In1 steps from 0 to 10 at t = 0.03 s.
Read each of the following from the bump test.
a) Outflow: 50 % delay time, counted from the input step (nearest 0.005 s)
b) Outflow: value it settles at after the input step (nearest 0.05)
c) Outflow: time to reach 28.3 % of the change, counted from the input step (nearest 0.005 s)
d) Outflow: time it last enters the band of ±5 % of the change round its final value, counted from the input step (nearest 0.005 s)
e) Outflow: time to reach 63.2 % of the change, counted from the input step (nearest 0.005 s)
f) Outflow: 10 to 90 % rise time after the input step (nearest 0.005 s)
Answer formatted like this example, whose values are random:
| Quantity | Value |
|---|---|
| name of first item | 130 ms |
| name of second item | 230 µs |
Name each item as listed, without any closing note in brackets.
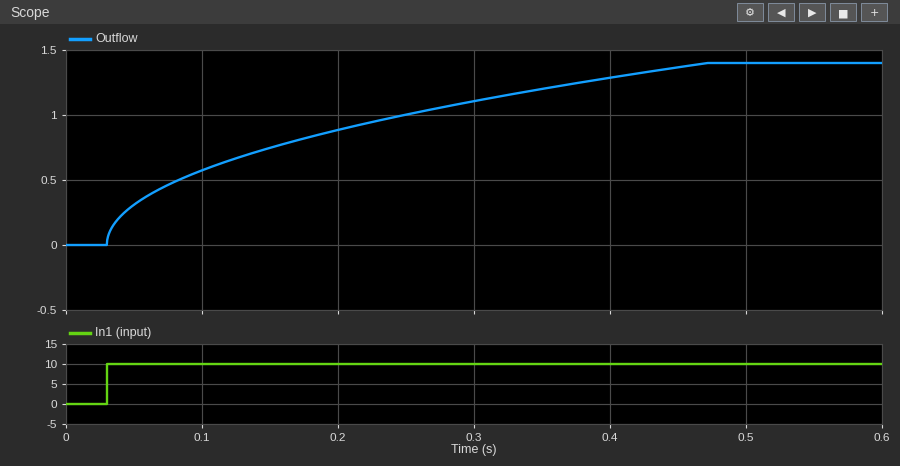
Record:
| Quantity | Value |
|---|---|
| Outflow: 50 % delay time, counted from the input step | 0.105 s |
| Outflow: value it settles at after the input step | 1.40 |
| Outflow: time to reach 28.3 % of the change, counted from the input step | 0.035 s |
| Outflow: time it last enters the band of ±5 % of the change round its final value, counted from the input step | 0.395 s |
| Outflow: time to reach 63.2 % of the change, counted from the input step | 0.170 s |
| Outflow: 10 to 90 % rise time after the input step | 0.350 s |
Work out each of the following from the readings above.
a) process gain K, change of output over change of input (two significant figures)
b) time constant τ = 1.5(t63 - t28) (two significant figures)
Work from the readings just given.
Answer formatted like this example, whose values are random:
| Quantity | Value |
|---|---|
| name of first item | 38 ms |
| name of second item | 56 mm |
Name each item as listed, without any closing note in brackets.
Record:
| Quantity | Value |
|---|---|
| process gain K, change of output over change of input | 0.14 |
| time constant τ = 1.5(t63 - t28) | 0.20 s |
